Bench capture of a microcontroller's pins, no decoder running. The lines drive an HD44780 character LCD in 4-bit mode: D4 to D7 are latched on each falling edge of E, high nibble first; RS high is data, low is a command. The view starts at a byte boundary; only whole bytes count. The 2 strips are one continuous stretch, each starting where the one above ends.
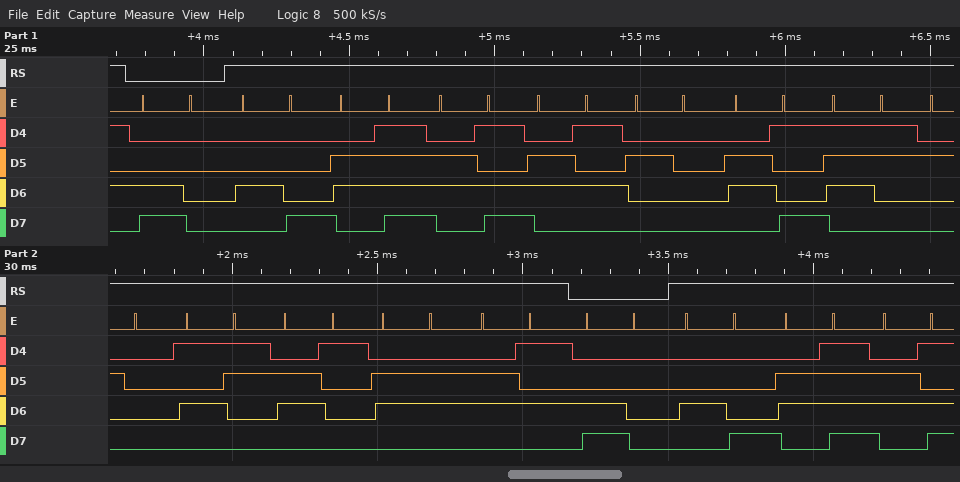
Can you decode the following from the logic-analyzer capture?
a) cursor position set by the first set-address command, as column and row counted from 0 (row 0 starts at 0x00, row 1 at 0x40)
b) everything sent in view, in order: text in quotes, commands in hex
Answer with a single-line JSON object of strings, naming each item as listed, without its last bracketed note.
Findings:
{"cursor position set by the first set-address command, as column and row counted from 0": "column 0, row 1", "everything sent in view, in order: text in quotes, commands in hex": "0xC0 \"Home is Safe\" 0xC0 \"Hom\""}
